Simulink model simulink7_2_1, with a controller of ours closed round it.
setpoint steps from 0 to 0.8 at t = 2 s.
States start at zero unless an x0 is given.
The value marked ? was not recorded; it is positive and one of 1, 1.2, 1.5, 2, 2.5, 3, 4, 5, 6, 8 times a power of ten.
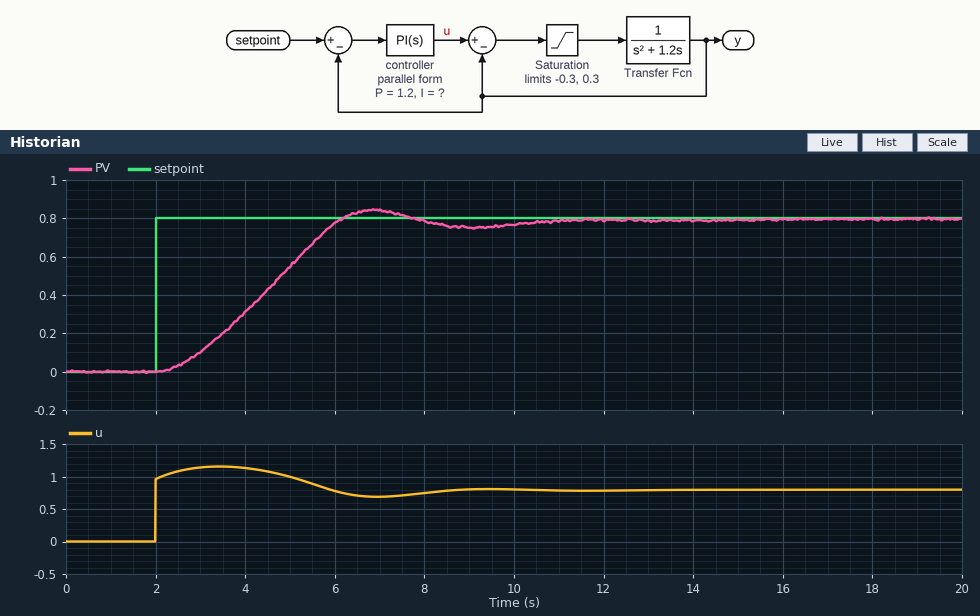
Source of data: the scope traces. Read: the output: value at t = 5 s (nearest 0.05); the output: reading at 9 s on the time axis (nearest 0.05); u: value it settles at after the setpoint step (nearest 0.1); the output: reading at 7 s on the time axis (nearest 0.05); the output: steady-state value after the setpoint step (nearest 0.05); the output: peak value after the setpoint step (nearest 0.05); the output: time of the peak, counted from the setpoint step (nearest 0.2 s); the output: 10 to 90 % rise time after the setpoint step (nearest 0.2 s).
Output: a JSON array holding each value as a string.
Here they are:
["0.55", "0.75", "0.8", "0.85", "0.80", "0.85", "4.8 s", "2.8 s"]
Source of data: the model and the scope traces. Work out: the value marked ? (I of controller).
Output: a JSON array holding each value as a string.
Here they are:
["0.4"]
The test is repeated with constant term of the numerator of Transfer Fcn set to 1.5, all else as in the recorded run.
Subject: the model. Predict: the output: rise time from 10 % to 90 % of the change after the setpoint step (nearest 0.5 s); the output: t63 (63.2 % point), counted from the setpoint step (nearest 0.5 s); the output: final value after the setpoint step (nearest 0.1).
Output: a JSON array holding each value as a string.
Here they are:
["2.0 s", "2.0 s", "0.8"]
